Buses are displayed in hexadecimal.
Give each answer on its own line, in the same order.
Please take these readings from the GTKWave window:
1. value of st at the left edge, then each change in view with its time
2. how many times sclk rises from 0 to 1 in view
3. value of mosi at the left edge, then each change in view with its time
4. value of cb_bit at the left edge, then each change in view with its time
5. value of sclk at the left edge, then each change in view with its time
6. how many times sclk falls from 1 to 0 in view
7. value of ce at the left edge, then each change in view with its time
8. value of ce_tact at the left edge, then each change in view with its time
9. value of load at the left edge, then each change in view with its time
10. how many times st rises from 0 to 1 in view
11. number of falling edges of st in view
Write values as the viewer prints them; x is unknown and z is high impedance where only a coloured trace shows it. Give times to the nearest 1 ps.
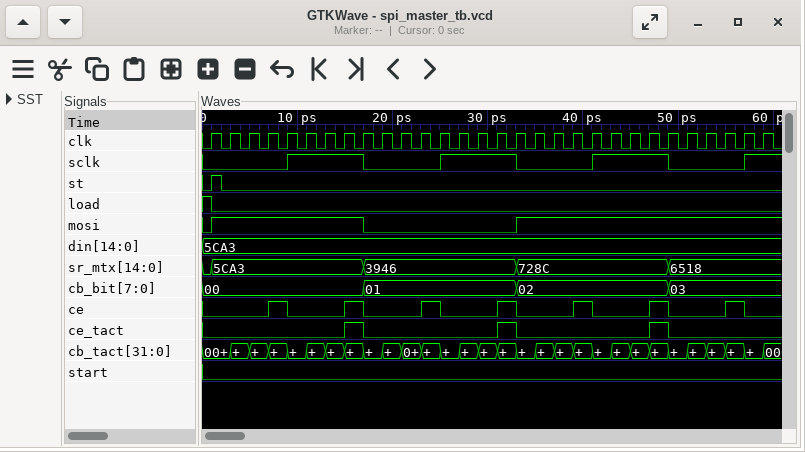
0, 1 at 1 ps, 0 at 2 ps
4
0, 1 at 1 ps, 0 at 17 ps, 1 at 33 ps
00, 01 at 17 ps, 02 at 33 ps, 03 at 49 ps
0, 1 at 9 ps, 0 at 17 ps, 1 at 25 ps, 0 at 33 ps, 1 at 41 ps, 0 at 49 ps, 1 at 57 ps
3
0, 1 at 7 ps, 0 at 9 ps, 1 at 15 ps, 0 at 17 ps, 1 at 23 ps, 0 at 25 ps, 1 at 31 ps, 0 at 33 ps, 1 at 39 ps, 0 at 41 ps, 1 at 47 ps, 0 at 49 ps, 1 at 55 ps, 0 at 57 ps
0, 1 at 15 ps, 0 at 17 ps, 1 at 31 ps, 0 at 33 ps, 1 at 47 ps, 0 at 49 ps
1, 0 at 1 ps
1
1
